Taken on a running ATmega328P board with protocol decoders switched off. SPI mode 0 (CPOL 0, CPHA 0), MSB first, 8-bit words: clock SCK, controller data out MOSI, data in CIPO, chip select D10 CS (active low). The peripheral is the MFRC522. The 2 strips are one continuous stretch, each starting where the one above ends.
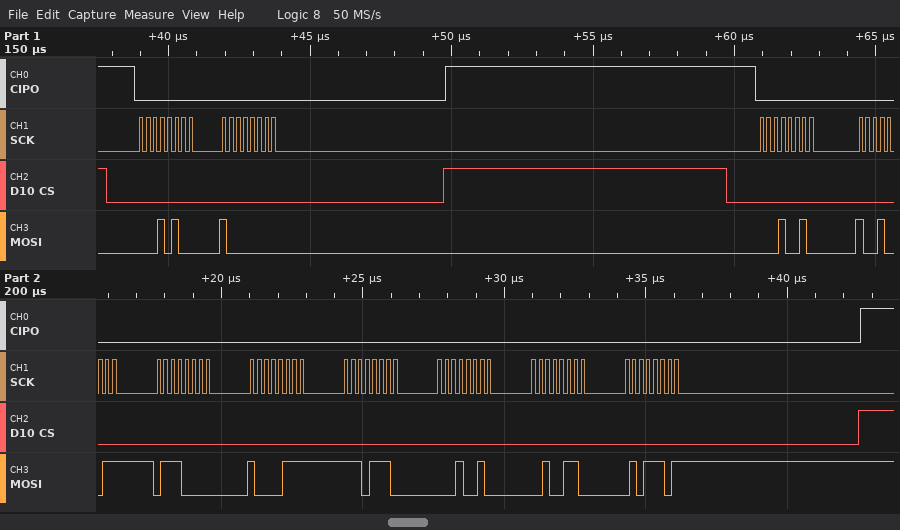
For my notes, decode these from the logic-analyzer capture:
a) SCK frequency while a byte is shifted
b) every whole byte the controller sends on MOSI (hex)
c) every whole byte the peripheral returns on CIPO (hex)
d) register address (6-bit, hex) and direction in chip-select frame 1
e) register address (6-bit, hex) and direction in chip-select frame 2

4 MHz
14 80 12 93 70 87 EE 12 26 5D
00 00 00 00 00 00 00 00 00 00
0x0A write
0x09 write
